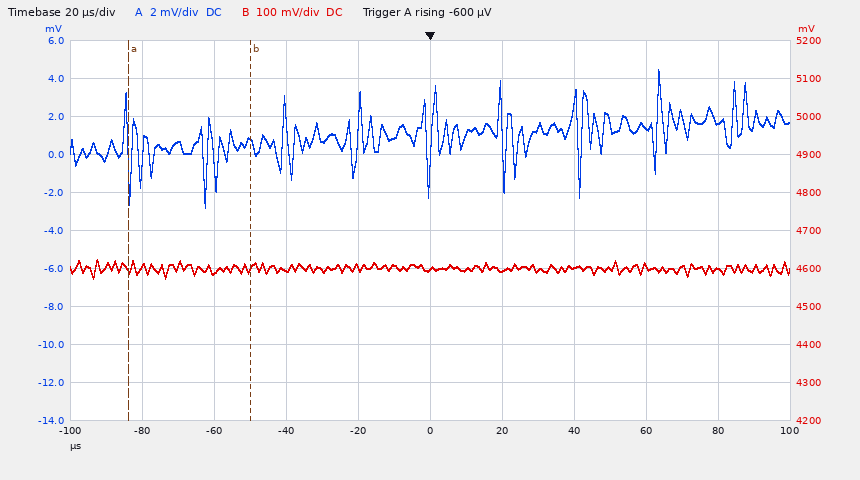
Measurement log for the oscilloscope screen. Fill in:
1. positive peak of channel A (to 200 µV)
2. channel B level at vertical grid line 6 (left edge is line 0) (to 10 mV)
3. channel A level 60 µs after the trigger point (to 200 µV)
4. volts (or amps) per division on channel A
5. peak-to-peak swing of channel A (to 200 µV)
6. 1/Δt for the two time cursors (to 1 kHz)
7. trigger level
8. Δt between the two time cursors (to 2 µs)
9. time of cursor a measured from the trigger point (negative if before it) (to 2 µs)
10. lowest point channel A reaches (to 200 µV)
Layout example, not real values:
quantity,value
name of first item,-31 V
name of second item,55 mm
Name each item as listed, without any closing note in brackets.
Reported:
quantity,value
positive peak of channel A,4.4 mV
channel B level at vertical grid line 6 (left edge is line 0),4.59 V
channel A level 60 µs after the trigger point,1.4 mV
volts (or amps) per division on channel A,2 mV
peak-to-peak swing of channel A,7.2 mV
1/Δt for the two time cursors,29 kHz
trigger level,-600 µV
Δt between the two time cursors,34 µs
time of cursor a measured from the trigger point (negative if before it),-84 µs
lowest point channel A reaches,-2.8 mV
